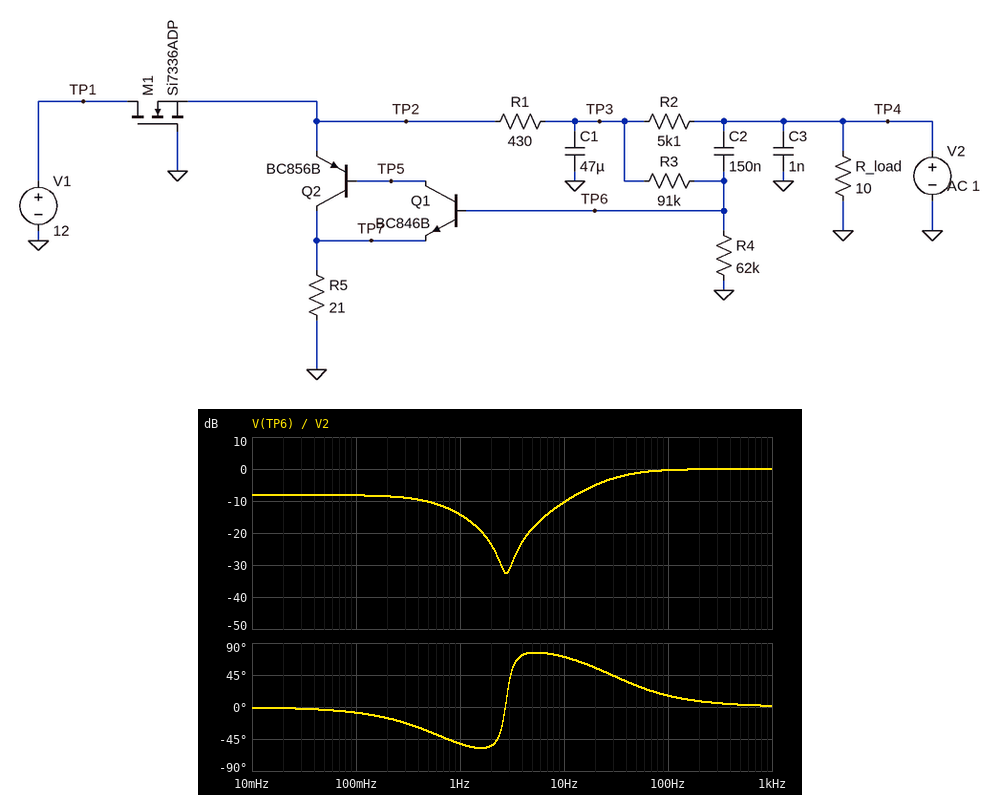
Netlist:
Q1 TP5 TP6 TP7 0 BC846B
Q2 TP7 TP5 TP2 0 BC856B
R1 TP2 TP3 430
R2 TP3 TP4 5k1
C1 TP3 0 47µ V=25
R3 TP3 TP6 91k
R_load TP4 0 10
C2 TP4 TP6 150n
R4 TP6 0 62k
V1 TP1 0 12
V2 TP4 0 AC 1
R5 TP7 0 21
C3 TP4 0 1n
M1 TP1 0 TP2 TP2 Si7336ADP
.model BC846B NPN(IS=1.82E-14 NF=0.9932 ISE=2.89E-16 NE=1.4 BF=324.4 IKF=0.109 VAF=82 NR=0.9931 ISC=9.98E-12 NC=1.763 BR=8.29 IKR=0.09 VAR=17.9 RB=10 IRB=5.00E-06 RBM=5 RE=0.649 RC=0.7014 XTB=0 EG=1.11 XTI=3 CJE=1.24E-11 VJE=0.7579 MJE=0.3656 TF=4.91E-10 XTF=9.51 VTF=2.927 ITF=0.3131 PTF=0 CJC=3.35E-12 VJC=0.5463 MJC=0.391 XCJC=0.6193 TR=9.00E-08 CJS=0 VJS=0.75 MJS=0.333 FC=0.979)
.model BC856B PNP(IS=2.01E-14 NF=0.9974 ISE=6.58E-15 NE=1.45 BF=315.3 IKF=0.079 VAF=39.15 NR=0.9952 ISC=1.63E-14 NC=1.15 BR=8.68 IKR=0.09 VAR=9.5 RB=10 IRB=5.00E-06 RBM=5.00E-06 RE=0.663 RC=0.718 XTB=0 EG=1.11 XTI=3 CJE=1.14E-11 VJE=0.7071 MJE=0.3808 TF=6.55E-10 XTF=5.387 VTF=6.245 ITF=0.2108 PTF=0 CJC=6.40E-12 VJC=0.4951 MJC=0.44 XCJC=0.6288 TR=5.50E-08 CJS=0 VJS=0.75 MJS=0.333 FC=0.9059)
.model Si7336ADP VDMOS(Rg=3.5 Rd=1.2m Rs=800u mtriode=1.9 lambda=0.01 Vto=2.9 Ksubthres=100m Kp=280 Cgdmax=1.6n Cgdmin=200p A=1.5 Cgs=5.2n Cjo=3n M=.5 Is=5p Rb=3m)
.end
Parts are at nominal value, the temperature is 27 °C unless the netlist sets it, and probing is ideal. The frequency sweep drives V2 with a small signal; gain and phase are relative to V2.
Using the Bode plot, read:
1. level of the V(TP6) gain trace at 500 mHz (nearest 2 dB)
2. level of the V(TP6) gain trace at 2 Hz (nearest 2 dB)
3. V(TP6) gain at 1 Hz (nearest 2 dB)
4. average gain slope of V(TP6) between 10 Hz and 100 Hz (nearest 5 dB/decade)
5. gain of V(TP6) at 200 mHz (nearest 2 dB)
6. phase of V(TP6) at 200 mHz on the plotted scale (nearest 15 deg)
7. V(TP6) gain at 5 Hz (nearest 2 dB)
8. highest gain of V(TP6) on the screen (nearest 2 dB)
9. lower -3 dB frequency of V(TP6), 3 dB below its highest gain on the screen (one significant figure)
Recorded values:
-10 dB
-24 dB
-14 dB
10 dB/decade
-8 dB
-15 deg
-18 dB
0 dB
30 Hz
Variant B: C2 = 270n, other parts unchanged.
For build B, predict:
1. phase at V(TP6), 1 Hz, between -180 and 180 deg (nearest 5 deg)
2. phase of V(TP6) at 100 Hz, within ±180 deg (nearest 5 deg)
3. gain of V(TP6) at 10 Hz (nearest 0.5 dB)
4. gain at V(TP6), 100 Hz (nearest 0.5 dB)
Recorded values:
-45 deg
10 deg
-6.0 dB
0 dB
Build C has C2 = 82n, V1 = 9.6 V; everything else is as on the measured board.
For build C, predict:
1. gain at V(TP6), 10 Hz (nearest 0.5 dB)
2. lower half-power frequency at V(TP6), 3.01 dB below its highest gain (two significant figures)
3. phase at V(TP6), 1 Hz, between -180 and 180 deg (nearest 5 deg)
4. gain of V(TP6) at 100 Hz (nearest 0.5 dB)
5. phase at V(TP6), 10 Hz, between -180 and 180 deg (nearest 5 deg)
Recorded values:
-16.0 dB
53 Hz
-55 deg
-1.0 dB
80 deg
